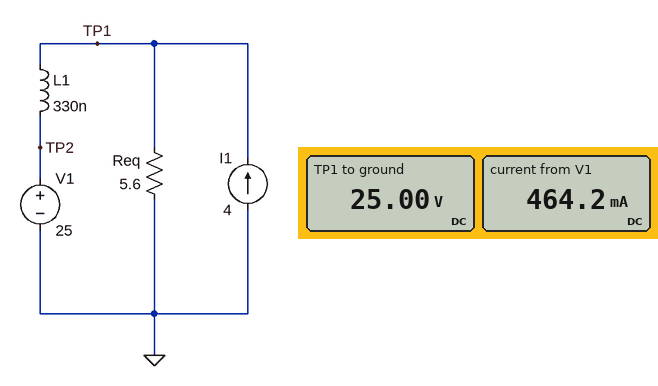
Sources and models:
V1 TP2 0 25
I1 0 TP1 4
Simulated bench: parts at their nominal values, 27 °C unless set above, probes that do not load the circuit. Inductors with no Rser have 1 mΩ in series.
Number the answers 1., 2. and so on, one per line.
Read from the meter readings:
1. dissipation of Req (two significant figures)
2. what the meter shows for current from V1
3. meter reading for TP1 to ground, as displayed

1. 110 W
2. 464.2 mA
3. 25.00 V
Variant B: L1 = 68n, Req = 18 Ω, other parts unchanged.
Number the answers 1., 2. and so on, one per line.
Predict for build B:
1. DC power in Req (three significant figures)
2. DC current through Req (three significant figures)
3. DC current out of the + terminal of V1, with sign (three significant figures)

1. 34.7 W
2. 1.39 A
3. -2.61 A
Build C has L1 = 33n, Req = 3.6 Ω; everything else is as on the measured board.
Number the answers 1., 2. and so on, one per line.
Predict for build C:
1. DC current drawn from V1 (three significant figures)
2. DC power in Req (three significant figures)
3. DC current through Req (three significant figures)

1. 2.94 A
2. 174 W
3. 6.94 A
